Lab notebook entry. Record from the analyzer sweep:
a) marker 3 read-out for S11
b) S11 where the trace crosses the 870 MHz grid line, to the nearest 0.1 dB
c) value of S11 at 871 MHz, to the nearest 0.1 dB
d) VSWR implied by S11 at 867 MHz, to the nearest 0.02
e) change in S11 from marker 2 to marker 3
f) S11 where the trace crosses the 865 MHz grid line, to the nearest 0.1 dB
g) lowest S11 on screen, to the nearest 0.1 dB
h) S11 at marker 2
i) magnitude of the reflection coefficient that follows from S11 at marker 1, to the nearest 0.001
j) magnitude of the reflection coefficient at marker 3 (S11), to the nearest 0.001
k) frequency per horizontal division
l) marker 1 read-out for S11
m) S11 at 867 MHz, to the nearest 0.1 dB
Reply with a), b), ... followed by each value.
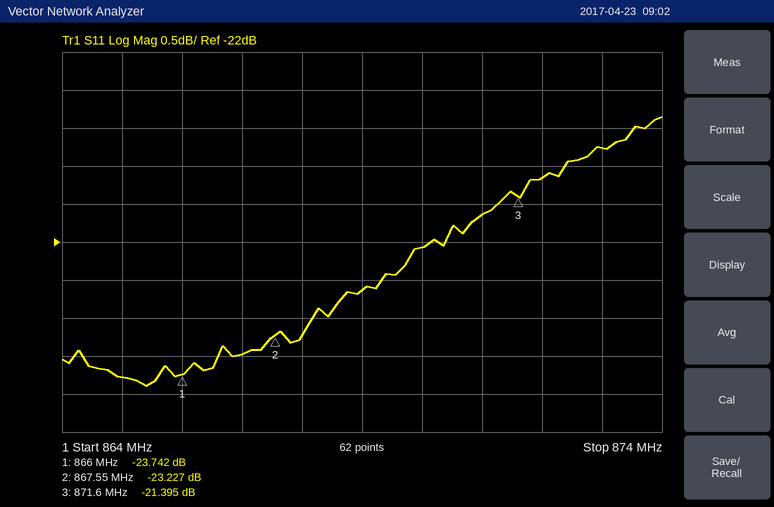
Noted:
a) -21.395 dB
b) -22.1 dB
c) -21.6 dB
d) 1.14
e) 1.832 dB
f) -23.8 dB
g) -23.9 dB
h) -23.227 dB
i) 0.065
j) 0.085
k) 1 MHz
l) -23.742 dB
m) -23.5 dB
